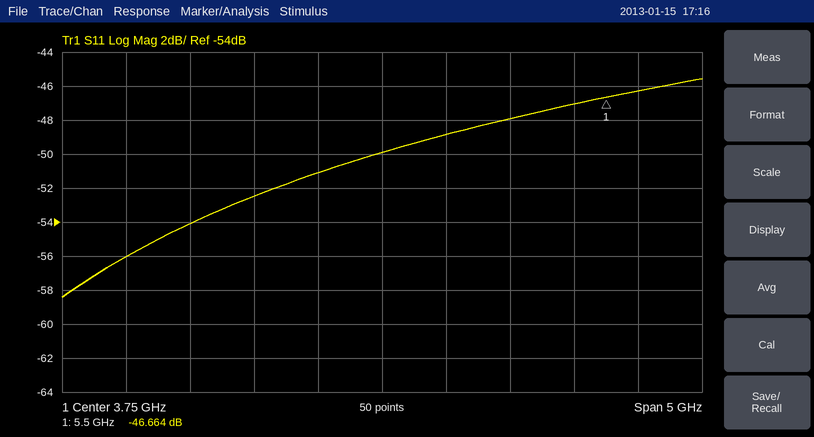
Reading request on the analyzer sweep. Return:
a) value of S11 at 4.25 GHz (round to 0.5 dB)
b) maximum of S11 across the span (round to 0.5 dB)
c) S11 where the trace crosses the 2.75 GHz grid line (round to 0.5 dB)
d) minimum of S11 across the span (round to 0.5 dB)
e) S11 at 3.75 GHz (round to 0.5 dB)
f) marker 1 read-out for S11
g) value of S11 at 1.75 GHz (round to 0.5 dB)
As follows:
-49.0 dB
-45.5 dB
-52.5 dB
-58.5 dB
-50.0 dB
-46.664 dB
-56.0 dB
